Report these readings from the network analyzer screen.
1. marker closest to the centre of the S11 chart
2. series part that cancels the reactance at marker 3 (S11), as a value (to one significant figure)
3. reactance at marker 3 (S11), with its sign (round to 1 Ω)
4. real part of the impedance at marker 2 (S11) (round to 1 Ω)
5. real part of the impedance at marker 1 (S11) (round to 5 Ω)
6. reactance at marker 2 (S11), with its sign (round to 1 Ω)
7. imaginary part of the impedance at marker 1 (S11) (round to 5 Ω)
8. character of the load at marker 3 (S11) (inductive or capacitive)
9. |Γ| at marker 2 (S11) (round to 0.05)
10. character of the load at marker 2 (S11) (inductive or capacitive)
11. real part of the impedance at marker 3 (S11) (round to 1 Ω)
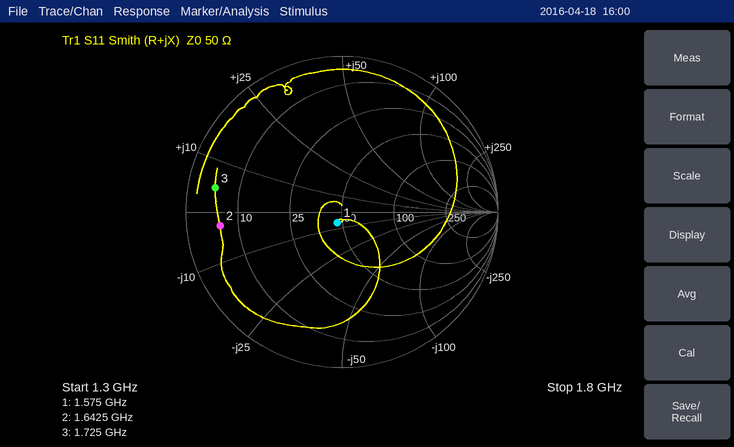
marker 1
20 pF
+5 Ω
6 Ω
45 Ω
-3 Ω
-5 Ω
inductive
0.80
capacitive
5 Ω
